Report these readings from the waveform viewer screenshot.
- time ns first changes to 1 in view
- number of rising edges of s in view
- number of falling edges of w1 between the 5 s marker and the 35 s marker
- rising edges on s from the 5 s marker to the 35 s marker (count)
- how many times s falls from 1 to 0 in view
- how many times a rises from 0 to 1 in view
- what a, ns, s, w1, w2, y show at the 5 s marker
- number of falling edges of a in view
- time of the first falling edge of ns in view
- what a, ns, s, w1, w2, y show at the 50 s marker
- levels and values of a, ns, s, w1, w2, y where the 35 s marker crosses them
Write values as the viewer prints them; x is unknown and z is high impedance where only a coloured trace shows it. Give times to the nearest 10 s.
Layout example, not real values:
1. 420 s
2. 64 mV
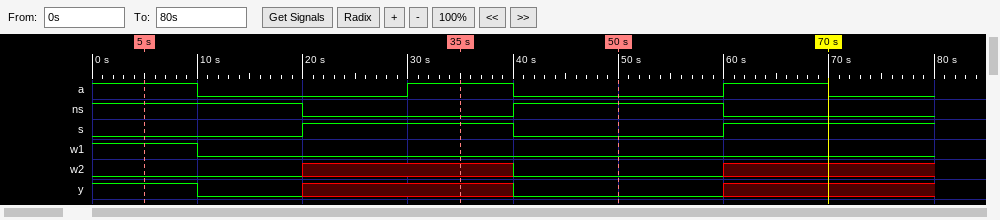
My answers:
1. 40 s
2. 2
3. 1
4. 1
5. 1
6. 2
7. a=1, ns=1, s=0, w1=1, w2=0, y=1
8. 3
9. 20 s
10. a=0, ns=1, s=0, w1=0, w2=0, y=0
11. a=1, ns=0, s=1, w1=0, w2=x, y=x
